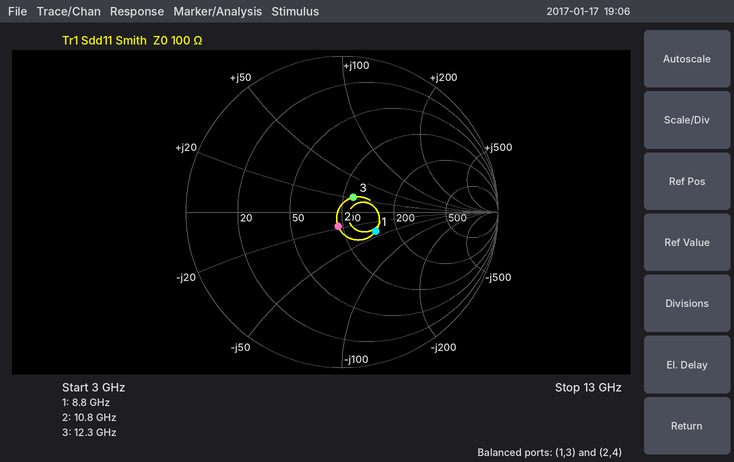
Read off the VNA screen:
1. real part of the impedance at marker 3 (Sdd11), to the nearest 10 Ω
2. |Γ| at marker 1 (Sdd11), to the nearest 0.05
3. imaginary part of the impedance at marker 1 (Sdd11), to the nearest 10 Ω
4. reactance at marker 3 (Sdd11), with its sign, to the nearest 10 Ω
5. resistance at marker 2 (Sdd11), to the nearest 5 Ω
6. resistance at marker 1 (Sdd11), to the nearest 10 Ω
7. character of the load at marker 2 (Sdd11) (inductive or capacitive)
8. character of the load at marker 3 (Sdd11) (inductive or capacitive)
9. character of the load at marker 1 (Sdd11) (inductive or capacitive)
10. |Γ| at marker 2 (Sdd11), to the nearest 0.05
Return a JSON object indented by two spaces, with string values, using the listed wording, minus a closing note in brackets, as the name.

{
  "real part of the impedance at marker 3 (Sdd11), to the nearest 10 Ω": "110 Ω",
  "|Γ| at marker 1 (Sdd11), to the nearest 0.05": "0.25",
  "imaginary part of the impedance at marker 1 (Sdd11), to the nearest 10 Ω": "-40 Ω",
  "reactance at marker 3 (Sdd11), with its sign, to the nearest 10 Ω": "+20 Ω",
  "resistance at marker 2 (Sdd11), to the nearest 5 Ω": "95 Ω",
  "resistance at marker 1 (Sdd11), to the nearest 10 Ω": "150 Ω",
  "character of the load at marker 2 (Sdd11)": "capacitive",
  "character of the load at marker 3 (Sdd11)": "inductive",
  "character of the load at marker 1 (Sdd11)": "capacitive",
  "|Γ| at marker 2 (Sdd11), to the nearest 0.05": "0.10"
}
